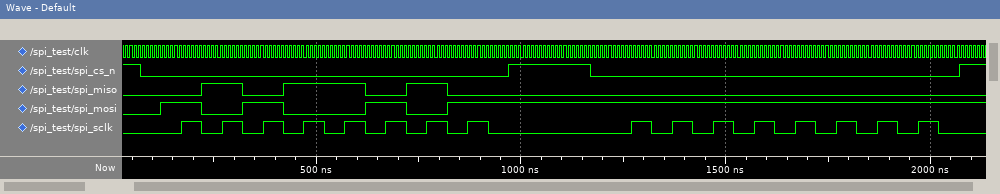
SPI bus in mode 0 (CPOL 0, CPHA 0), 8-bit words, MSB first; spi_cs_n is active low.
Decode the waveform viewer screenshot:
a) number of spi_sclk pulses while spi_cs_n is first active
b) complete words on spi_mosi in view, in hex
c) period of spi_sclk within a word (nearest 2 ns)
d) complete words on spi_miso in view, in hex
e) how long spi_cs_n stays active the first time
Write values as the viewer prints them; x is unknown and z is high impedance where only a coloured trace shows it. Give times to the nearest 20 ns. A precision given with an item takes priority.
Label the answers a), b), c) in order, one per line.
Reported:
a) 8
b) A5, FF
c) 100 ns
d) 5A, 00
e) 900 ns
